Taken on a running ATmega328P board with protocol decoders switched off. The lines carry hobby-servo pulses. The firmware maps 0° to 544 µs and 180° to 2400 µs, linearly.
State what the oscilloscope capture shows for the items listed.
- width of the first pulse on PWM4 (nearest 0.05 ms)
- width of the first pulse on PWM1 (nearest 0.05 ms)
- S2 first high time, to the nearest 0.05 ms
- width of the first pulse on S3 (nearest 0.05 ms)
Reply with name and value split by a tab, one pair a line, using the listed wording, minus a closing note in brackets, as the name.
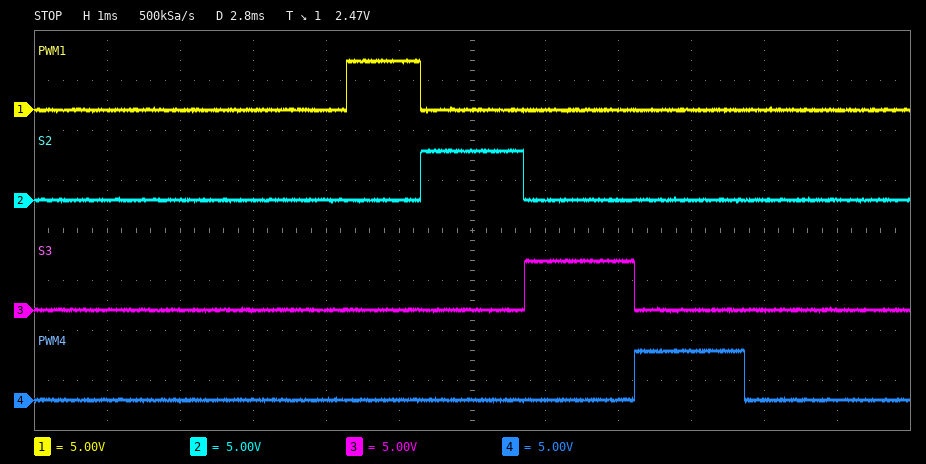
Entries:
width of the first pulse on PWM4	1.50 ms
width of the first pulse on PWM1	1.00 ms
S2 first high time, to the nearest 0.05 ms	1.40 ms
width of the first pulse on S3	1.50 ms
